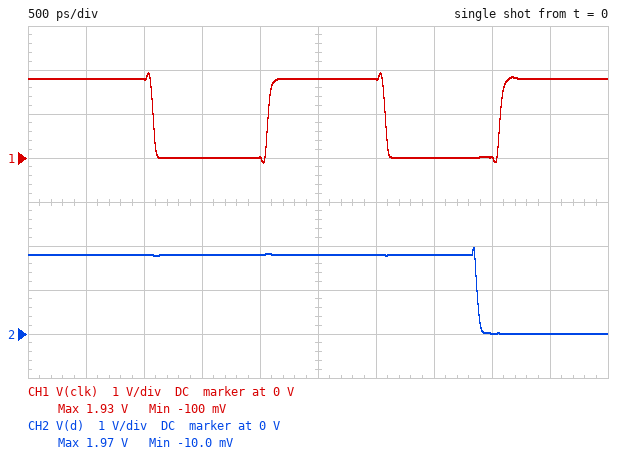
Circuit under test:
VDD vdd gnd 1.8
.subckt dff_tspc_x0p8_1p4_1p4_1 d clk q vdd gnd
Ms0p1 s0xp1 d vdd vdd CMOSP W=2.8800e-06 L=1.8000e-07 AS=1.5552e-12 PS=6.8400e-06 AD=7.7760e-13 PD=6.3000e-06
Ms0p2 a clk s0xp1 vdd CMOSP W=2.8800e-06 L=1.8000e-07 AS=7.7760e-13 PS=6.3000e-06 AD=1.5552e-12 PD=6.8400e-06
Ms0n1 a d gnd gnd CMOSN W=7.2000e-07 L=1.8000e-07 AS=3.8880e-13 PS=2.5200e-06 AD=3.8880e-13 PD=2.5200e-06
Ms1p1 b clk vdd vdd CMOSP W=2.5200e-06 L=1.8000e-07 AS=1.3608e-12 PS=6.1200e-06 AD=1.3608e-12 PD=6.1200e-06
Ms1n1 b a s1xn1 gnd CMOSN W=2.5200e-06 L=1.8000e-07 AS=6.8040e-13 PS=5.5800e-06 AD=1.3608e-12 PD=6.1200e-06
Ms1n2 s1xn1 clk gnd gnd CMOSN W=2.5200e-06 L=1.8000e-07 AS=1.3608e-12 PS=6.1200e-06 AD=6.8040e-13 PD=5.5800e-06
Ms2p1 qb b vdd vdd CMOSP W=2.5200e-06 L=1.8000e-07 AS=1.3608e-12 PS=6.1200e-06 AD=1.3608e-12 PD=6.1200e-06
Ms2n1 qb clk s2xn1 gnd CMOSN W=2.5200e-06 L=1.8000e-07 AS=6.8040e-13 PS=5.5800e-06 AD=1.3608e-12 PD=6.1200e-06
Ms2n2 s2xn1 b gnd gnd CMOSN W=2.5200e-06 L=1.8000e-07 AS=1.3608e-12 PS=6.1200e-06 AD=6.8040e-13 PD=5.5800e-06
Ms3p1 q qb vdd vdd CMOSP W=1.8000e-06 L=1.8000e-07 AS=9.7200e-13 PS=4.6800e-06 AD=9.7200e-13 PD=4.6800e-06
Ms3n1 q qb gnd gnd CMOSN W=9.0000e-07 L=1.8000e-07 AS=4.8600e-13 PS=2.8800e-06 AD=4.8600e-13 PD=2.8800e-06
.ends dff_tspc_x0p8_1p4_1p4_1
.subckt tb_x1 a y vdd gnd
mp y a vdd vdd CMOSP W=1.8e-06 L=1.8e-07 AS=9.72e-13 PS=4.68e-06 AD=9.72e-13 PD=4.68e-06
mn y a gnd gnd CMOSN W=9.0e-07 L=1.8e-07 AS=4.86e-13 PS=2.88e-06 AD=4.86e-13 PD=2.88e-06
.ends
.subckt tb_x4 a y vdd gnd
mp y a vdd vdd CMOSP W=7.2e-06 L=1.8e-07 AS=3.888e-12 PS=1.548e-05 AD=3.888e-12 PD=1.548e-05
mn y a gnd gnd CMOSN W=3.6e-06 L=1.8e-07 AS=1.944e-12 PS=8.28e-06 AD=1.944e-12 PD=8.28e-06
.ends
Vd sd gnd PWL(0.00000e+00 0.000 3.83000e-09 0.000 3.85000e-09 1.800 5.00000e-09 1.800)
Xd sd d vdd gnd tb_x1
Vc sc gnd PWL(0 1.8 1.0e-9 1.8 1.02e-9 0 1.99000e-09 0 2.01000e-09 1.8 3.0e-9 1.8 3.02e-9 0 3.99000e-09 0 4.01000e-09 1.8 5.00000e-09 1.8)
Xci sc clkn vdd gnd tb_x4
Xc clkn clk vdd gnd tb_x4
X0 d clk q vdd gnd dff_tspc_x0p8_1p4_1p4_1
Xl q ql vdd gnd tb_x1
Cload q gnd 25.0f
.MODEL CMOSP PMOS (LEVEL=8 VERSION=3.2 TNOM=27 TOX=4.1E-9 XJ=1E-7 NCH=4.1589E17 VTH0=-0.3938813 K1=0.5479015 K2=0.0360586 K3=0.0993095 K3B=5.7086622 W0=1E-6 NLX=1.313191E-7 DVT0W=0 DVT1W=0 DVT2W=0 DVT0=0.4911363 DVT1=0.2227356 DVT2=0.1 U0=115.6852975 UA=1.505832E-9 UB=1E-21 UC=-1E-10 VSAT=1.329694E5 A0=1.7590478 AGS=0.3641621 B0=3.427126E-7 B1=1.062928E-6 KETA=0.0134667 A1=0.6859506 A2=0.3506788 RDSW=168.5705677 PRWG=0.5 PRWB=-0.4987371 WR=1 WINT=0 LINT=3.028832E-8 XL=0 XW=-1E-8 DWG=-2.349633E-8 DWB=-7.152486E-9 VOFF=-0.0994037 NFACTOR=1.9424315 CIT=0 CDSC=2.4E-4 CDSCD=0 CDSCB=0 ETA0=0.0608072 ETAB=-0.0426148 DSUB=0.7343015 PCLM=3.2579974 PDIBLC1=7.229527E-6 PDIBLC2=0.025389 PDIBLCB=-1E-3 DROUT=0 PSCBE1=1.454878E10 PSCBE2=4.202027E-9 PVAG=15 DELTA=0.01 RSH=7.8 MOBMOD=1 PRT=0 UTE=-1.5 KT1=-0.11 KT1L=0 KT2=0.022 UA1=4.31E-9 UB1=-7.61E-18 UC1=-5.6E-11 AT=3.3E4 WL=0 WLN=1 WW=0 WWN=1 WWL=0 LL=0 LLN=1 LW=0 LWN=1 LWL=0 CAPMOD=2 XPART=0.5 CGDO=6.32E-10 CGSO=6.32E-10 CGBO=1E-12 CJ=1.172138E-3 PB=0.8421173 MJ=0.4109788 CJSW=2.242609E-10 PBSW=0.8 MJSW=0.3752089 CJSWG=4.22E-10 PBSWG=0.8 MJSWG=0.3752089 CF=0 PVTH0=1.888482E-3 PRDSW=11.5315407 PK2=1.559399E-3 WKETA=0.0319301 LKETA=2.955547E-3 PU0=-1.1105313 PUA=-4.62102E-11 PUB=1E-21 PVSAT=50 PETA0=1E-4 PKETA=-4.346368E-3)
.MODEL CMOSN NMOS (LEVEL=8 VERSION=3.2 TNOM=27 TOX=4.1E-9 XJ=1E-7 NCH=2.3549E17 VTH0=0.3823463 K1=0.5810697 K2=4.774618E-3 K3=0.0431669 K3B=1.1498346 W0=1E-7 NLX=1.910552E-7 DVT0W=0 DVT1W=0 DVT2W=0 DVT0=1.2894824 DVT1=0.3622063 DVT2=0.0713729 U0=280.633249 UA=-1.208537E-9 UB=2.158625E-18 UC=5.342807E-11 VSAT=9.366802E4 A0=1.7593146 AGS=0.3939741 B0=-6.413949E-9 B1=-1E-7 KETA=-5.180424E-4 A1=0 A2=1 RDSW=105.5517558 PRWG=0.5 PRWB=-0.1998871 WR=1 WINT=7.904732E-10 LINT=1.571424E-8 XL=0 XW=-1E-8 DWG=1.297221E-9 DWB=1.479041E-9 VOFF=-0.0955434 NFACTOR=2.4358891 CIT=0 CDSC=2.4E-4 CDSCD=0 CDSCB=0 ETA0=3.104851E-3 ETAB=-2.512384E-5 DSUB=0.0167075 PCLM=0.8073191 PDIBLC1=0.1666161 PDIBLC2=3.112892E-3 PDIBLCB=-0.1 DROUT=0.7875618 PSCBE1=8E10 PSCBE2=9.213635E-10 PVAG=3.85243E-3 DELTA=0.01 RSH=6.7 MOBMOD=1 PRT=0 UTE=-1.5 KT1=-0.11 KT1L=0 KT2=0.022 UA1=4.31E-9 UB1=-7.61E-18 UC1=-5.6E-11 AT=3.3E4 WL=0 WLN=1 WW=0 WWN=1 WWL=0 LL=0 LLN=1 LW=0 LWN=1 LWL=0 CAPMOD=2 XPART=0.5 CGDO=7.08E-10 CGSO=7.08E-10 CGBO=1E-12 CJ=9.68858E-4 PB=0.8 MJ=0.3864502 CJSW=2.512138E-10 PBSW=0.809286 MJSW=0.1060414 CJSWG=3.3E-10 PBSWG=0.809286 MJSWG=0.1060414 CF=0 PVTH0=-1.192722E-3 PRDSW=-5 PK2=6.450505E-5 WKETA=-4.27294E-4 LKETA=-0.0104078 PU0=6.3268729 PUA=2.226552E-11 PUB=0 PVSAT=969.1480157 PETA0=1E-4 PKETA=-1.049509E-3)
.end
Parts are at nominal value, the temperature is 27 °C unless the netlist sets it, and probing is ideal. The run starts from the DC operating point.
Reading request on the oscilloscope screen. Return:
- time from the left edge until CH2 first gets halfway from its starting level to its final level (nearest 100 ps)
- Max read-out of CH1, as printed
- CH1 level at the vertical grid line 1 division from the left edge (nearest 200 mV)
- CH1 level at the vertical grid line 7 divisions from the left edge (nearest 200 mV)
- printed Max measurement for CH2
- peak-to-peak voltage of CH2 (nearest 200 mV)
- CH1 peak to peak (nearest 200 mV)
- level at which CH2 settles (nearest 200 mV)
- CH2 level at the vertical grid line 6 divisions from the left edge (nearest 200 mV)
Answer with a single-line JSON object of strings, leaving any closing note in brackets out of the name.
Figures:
{"time from the left edge until CH2 first gets halfway from its starting level to its final level": "3.9 ns", "Max read-out of CH1, as printed": "1.93 V", "CH1 level at the vertical grid line 1 division from the left edge": "1.8 V", "CH1 level at the vertical grid line 7 divisions from the left edge": "0 V", "printed Max measurement for CH2": "1.97 V", "peak-to-peak voltage of CH2": "2.0 V", "CH1 peak to peak": "2.0 V", "level at which CH2 settles": "0 V", "CH2 level at the vertical grid line 6 divisions from the left edge": "1.8 V"}
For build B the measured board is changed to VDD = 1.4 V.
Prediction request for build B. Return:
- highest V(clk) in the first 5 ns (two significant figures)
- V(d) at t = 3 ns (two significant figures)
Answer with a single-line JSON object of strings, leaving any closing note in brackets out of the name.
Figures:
{"highest V(clk) in the first 5 ns": "1.5 V", "V(d) at t = 3 ns": "1.4 V"}
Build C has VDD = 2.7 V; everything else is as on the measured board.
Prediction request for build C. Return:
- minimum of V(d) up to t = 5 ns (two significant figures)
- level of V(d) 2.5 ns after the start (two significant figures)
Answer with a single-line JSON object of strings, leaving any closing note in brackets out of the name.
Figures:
{"minimum of V(d) up to t = 5 ns": "54 mV", "level of V(d) 2.5 ns after the start": "2.7 V"}
